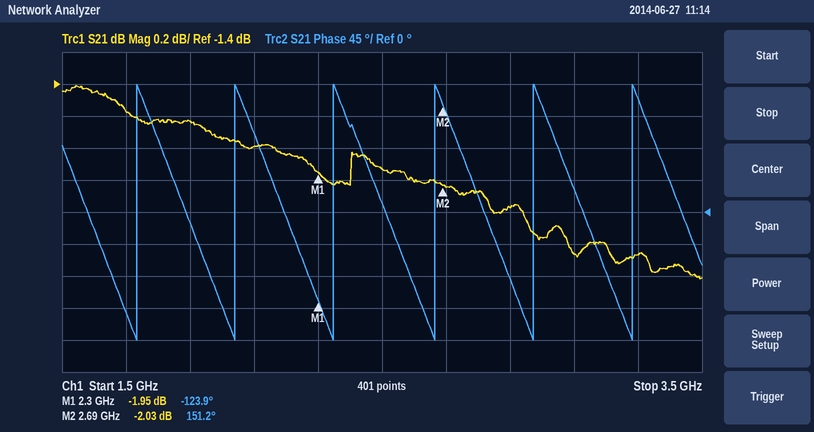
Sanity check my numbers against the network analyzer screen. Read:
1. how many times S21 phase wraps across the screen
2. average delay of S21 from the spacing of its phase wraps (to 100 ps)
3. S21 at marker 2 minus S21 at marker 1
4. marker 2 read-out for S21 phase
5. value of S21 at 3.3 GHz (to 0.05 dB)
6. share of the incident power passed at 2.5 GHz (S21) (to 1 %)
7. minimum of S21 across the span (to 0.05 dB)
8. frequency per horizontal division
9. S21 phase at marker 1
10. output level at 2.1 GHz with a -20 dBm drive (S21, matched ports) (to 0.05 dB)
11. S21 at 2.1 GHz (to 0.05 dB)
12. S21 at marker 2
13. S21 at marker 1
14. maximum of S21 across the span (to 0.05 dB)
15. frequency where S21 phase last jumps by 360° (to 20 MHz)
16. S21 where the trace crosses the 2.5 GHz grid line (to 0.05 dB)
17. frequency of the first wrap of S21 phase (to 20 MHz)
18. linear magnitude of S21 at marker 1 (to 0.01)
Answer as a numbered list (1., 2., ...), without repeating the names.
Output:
1. 6
2. 3.2 ns
3. -0.08 dB
4. 151.2°
5. -2.45 dB
6. 64 %
7. -2.60 dB
8. 200 MHz
9. -123.9°
10. -21.80 dBm
11. -1.80 dB
12. -2.03 dB
13. -1.95 dB
14. -1.40 dB
15. 3.28 GHz
16. -1.95 dB
17. 1.74 GHz
18. 0.80
